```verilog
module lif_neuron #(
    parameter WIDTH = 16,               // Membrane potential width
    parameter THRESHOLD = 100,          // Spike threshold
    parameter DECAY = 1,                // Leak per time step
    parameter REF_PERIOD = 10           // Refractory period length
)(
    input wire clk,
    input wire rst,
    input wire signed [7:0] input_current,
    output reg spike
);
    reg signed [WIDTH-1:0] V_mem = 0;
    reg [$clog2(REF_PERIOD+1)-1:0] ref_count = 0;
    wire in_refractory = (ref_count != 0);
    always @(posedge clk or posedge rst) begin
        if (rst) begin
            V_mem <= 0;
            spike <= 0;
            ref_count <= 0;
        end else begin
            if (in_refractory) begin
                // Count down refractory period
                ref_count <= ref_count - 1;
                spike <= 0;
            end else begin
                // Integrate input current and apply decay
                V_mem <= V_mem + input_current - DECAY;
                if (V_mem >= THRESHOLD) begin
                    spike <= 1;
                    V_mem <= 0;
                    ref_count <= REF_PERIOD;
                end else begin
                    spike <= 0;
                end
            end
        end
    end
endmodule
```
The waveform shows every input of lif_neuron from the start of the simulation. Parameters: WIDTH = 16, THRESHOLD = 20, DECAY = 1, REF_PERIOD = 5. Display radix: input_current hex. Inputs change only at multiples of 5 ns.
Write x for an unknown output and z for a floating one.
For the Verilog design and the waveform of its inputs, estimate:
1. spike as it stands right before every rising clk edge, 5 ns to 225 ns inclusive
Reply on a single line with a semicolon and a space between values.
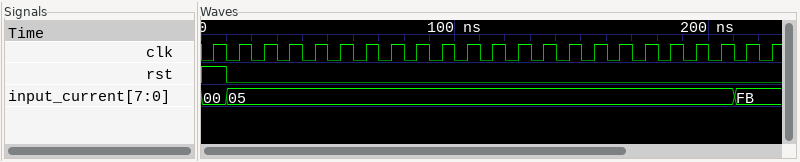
0 0 0 0 0 0 0 1 0 0 0 0 0 0 0 0 0 0 1 0 0 0 0
